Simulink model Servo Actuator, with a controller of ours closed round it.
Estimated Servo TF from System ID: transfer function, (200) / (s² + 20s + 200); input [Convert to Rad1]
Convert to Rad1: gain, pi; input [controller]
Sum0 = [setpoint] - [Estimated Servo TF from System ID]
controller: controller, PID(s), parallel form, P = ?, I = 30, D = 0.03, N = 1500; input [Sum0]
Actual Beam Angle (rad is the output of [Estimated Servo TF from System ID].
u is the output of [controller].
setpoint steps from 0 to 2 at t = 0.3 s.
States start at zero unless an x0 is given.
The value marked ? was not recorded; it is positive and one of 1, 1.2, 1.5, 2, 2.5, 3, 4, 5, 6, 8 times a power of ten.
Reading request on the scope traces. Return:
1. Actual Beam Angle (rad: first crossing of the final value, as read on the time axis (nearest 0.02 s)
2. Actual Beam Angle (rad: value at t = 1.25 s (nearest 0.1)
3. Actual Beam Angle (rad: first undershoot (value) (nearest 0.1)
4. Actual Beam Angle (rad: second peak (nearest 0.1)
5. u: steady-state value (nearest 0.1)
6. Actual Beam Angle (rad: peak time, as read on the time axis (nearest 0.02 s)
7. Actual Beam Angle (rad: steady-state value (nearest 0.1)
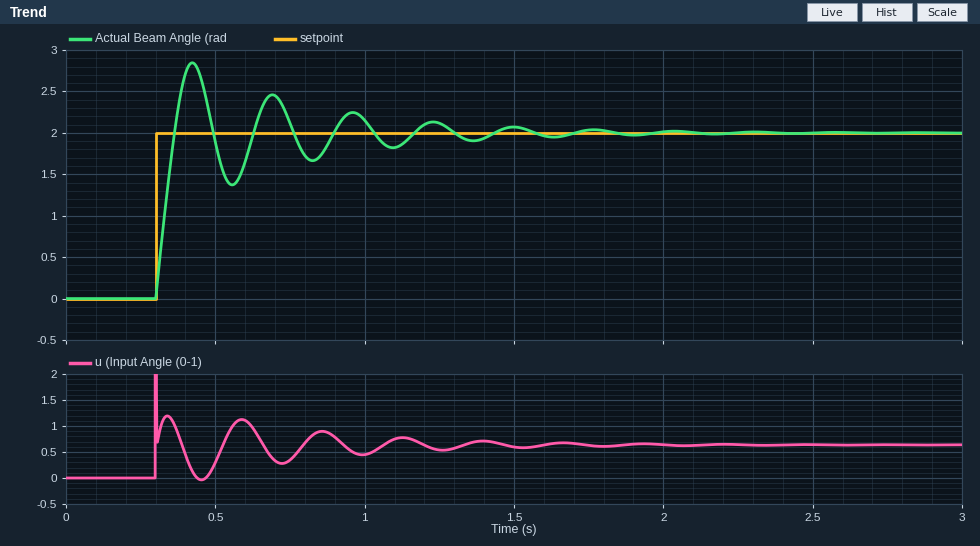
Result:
0.36 s
2.1
1.4
2.5
0.6
0.42 s
2.0
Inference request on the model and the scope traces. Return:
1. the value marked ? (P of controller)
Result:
0.8
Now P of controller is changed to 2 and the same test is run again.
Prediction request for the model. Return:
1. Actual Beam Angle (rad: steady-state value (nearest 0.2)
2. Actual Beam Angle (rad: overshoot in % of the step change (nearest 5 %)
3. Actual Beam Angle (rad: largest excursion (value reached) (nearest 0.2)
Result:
2.0
30 %
2.6
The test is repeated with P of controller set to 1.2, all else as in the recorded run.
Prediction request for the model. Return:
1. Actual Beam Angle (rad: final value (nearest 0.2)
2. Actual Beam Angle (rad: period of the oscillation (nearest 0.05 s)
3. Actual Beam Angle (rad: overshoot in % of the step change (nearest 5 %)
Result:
2.0
0.25 s
35 %
